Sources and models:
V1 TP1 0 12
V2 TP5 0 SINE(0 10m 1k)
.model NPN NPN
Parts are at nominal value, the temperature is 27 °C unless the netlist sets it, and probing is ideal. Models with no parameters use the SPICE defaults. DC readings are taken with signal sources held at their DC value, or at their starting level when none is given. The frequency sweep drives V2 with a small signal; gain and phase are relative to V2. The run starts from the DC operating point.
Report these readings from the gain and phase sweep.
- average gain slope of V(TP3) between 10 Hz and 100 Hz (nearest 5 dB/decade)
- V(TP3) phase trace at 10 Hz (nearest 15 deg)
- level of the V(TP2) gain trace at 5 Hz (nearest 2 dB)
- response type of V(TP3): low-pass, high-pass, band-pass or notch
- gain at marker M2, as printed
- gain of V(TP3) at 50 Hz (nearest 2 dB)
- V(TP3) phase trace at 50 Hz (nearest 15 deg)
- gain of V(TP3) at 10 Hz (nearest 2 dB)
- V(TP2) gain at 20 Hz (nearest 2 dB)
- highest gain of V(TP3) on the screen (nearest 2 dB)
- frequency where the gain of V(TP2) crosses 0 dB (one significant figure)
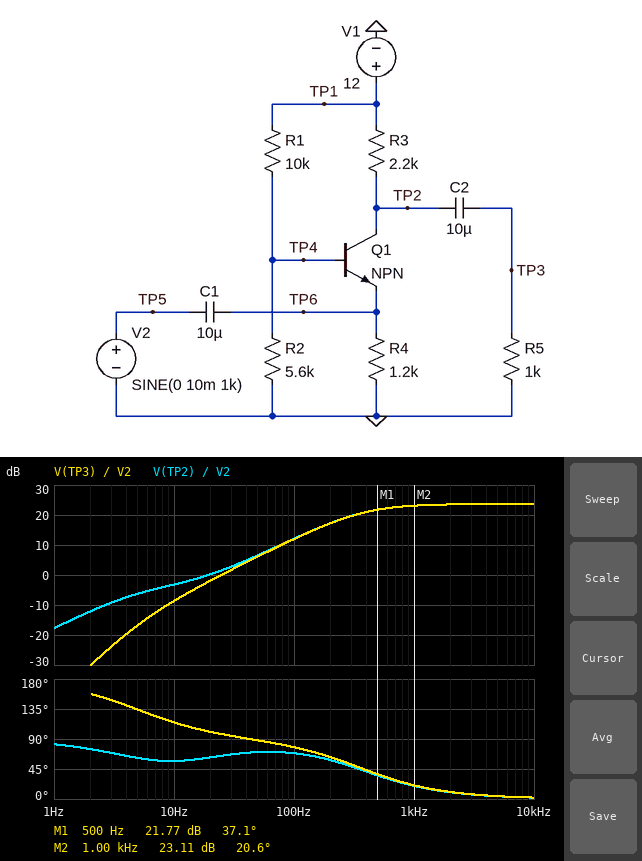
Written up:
20 dB/decade
120 deg
-6 dB
high-pass
23.11 dB
6 dB
90 deg
-8 dB
0 dB
24 dB
20 Hz
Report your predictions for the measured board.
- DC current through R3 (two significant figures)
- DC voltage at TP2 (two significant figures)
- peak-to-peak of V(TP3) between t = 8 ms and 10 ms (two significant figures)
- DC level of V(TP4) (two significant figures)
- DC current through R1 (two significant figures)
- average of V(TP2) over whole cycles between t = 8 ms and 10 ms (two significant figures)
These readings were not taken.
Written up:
2.8 mA
5.8 V
290 mV
4.2 V
780 µA
5.8 V
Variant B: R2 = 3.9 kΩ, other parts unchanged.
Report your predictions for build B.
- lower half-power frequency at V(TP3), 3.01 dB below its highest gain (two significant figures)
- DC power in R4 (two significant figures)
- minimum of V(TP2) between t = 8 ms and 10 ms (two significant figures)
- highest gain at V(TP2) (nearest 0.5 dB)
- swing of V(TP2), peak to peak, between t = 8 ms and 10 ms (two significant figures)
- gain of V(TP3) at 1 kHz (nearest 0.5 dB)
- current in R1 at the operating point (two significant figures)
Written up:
410 Hz
5.3 mW
7.3 V
24.5 dB
310 mV
24.0 dB
870 µA
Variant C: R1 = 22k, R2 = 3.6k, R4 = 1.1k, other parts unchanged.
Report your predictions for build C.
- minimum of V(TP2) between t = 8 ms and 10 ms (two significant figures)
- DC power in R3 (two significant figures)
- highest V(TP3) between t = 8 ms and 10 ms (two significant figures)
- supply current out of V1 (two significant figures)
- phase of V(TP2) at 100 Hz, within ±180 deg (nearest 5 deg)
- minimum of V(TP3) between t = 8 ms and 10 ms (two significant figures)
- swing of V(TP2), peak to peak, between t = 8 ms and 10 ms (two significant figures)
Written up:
10 V
1.4 mW
100 mV
1.3 mA
65 deg
-110 mV
210 mV
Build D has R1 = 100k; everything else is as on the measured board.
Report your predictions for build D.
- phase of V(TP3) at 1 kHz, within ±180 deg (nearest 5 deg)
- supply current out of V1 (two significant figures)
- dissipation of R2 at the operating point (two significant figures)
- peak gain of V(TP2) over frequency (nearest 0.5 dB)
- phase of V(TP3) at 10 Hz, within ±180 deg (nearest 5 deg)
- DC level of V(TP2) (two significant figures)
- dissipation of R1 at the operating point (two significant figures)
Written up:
0 deg
120 µA
72 µW
-19.5 dB
85 deg
12 V
1.3 mW
